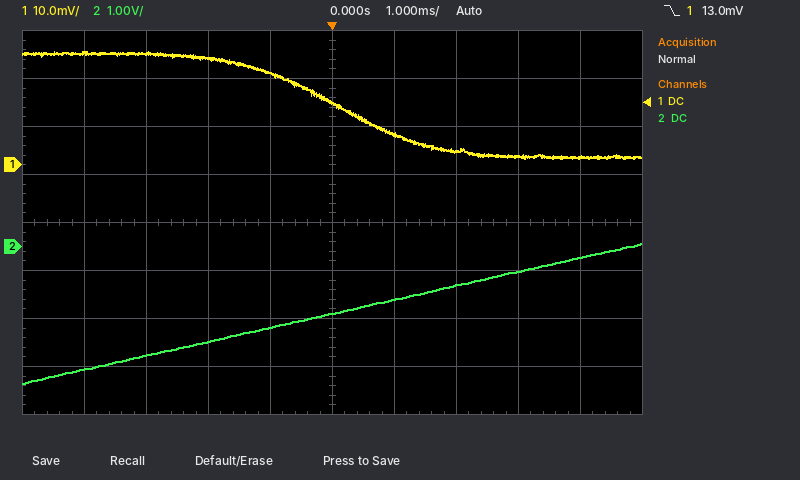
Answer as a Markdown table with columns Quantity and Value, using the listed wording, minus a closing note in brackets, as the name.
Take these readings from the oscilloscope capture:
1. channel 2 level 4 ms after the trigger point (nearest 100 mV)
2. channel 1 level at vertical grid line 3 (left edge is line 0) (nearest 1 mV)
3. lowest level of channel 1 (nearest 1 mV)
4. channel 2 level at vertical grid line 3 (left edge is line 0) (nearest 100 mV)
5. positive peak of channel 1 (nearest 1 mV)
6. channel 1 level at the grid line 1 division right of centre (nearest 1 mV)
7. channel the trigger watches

| Quantity | Value |
|---|---|
| channel 2 level 4 ms after the trigger point | -200 mV |
| channel 1 level at vertical grid line 3 (left edge is line 0) | 22 mV |
| lowest level of channel 1 | 1 mV |
| channel 2 level at vertical grid line 3 (left edge is line 0) | -2.0 V |
| positive peak of channel 1 | 24 mV |
| channel 1 level at the grid line 1 division right of centre | 6 mV |
| channel the trigger watches | channel 1 |
